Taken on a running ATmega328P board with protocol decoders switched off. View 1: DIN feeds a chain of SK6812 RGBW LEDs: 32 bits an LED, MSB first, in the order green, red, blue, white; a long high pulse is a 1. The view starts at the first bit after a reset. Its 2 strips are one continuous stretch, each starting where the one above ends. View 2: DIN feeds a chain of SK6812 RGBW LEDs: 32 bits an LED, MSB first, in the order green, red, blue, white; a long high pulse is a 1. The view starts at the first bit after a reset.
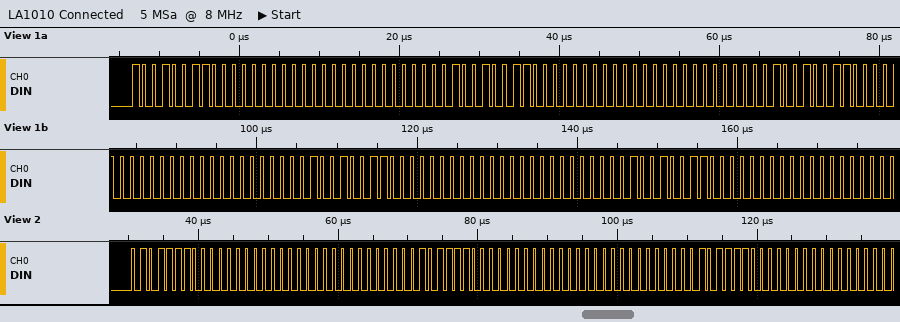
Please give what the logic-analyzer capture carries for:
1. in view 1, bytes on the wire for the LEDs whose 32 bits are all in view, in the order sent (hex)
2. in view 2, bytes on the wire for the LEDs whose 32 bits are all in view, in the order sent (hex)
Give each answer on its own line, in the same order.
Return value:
93 00 00 00 93 00 00 00 93 00 00 00 93 00 00 00
5E 00 00 00 5E 00 00 00
